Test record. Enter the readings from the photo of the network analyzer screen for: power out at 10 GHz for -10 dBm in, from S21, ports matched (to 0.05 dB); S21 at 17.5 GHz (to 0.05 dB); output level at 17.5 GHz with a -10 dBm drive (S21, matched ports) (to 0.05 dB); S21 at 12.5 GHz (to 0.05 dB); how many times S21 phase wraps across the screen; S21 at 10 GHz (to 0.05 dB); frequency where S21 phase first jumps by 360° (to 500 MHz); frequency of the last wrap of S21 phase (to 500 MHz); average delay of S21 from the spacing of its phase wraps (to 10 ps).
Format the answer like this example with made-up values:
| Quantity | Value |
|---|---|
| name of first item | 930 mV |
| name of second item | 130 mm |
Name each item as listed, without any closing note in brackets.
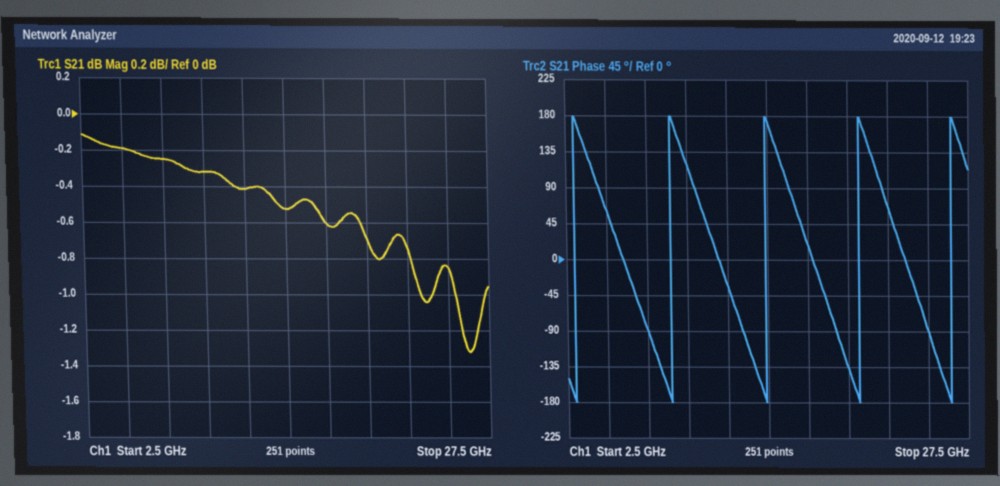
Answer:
| Quantity | Value |
|---|---|
| power out at 10 GHz for -10 dBm in, from S21, ports matched | -10.30 dBm |
| S21 at 17.5 GHz | -0.60 dB |
| output level at 17.5 GHz with a -10 dBm drive (S21, matched ports) | -10.60 dBm |
| S21 at 12.5 GHz | -0.40 dB |
| how many times S21 phase wraps across the screen | 5 |
| S21 at 10 GHz | -0.30 dB |
| frequency where S21 phase first jumps by 360° | 3.0 GHz |
| frequency of the last wrap of S21 phase | 26.5 GHz |
| average delay of S21 from the spacing of its phase wraps | 170 ps |
